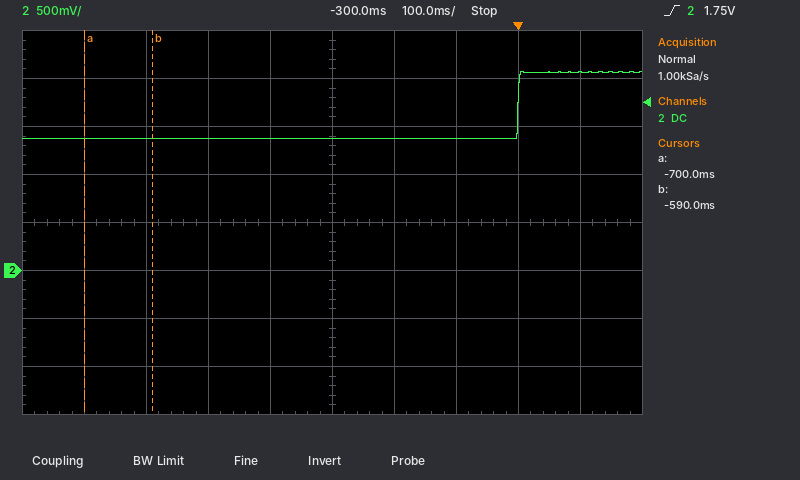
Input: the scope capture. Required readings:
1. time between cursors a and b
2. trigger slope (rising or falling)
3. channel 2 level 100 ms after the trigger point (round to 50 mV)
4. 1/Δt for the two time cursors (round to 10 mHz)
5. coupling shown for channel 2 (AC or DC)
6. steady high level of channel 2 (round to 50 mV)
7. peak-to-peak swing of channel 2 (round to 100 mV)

110 ms
rising
2.05 V
9.09 Hz
DC
2.05 V
700 mV
